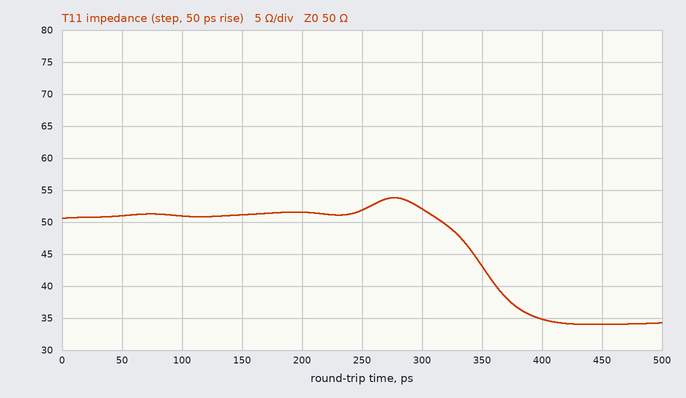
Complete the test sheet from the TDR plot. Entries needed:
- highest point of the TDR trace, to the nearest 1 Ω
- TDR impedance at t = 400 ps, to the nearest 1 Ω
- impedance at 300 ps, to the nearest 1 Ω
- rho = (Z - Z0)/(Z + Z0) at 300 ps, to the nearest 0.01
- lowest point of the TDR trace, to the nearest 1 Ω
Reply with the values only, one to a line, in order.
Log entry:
54 Ω
35 Ω
52 Ω
+0.02
34 Ω
